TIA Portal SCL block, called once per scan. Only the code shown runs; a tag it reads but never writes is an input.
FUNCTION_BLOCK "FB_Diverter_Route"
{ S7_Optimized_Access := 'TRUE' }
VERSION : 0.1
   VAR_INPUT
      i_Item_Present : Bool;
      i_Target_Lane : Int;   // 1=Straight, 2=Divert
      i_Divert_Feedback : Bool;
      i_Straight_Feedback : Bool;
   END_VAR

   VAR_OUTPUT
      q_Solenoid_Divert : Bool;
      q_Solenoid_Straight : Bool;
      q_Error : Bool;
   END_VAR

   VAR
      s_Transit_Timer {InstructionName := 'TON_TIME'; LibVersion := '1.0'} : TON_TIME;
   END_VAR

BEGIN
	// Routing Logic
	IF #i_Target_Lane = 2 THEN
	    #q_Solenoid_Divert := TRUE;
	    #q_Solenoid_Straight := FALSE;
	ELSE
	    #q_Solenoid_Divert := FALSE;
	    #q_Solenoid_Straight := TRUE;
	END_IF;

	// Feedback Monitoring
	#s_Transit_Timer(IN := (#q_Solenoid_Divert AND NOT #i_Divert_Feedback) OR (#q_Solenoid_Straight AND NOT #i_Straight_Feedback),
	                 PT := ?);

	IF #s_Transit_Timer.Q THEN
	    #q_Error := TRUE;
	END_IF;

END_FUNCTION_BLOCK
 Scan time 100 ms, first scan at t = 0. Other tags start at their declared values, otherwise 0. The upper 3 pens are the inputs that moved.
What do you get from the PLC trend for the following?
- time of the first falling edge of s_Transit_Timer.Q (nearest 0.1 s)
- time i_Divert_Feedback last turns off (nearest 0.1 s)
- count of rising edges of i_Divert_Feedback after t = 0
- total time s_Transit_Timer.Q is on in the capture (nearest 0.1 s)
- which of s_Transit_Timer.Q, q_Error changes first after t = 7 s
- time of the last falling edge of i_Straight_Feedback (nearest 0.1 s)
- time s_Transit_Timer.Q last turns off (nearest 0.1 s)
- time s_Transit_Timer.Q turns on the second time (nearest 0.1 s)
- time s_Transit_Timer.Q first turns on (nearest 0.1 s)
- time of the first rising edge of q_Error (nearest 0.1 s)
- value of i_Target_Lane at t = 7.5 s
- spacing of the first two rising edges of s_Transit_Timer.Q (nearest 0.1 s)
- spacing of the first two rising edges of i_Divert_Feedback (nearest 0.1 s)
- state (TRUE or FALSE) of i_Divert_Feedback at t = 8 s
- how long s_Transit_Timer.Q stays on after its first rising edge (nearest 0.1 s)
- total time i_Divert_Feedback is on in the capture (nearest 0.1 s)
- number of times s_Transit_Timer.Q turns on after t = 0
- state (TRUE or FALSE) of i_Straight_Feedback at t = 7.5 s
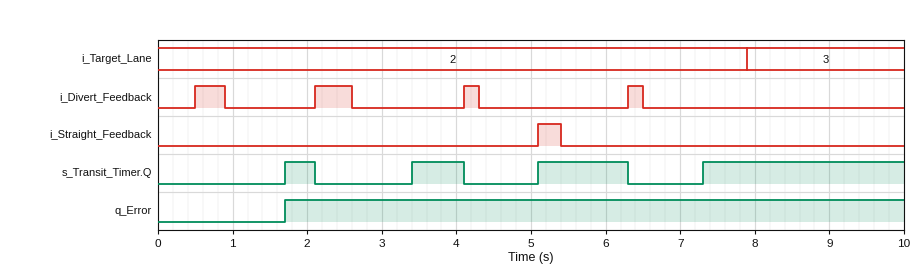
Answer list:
2.1 s
6.5 s
4
5.0 s
s_Transit_Timer.Q
5.4 s
6.3 s
3.4 s
1.7 s
1.7 s
2
1.7 s
1.6 s
FALSE
0.4 s
1.3 s
4
FALSE
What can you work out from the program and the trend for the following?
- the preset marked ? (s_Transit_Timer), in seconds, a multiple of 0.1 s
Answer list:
0.8 s
